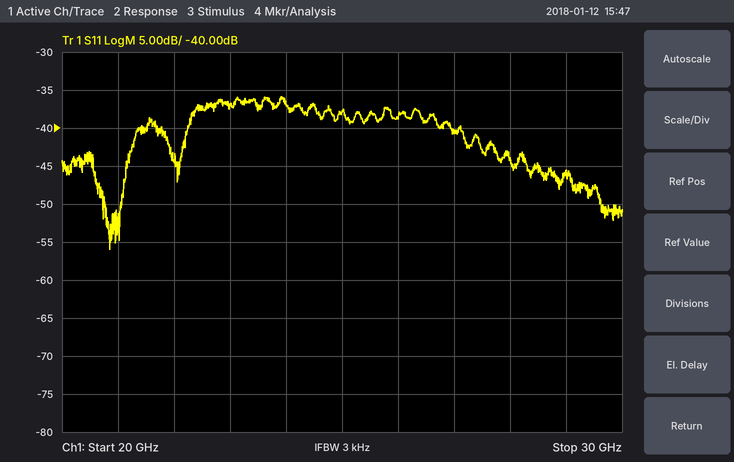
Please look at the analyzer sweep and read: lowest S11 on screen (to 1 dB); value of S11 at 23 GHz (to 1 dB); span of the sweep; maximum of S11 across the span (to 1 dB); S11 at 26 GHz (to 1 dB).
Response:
-56 dB
-37 dB
10 GHz
-36 dB
-39 dB
